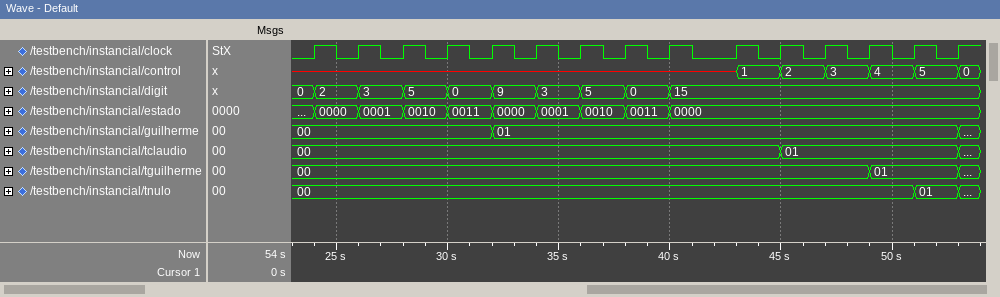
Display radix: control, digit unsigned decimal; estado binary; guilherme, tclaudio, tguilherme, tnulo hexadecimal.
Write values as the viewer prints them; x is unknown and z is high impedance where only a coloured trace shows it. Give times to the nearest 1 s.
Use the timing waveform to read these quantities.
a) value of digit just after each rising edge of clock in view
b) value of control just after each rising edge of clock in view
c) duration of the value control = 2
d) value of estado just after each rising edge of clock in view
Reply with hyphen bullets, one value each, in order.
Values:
- 2, 3, 5, 0, 9, 3, 5, 0, 15, 15, 15, 15, 15, 15, 15
- x, x, x, x, x, x, x, x, x, 1, 2, 3, 4, 5, 0
- 2 s
- 0000, 0001, 0010, 0011, 0000, 0001, 0010, 0011, 0000, 0000, 0000, 0000, 0000, 0000, 0000
